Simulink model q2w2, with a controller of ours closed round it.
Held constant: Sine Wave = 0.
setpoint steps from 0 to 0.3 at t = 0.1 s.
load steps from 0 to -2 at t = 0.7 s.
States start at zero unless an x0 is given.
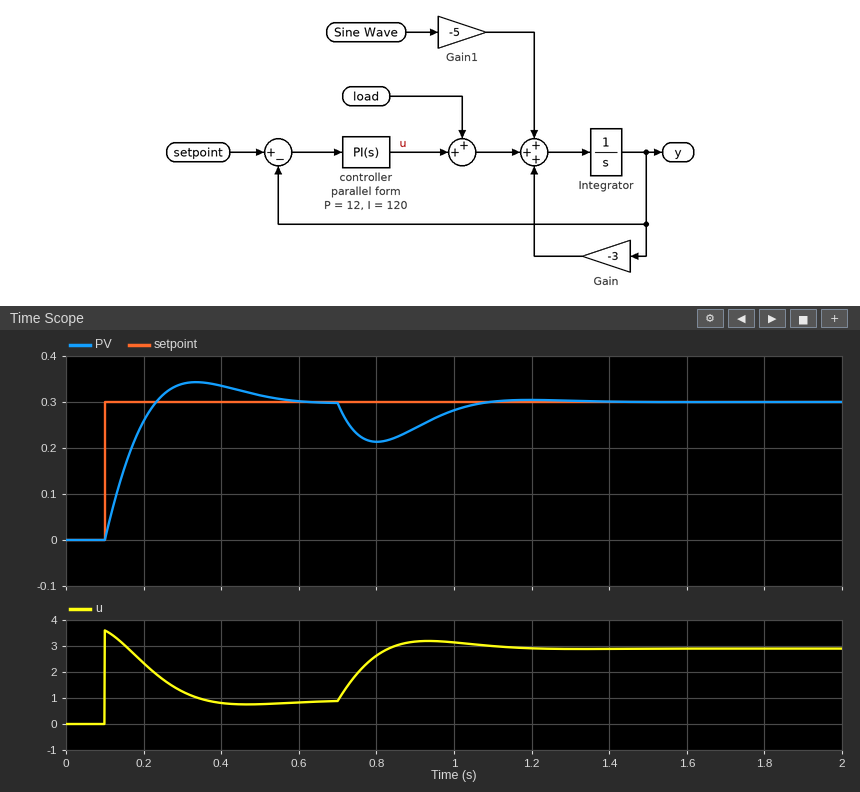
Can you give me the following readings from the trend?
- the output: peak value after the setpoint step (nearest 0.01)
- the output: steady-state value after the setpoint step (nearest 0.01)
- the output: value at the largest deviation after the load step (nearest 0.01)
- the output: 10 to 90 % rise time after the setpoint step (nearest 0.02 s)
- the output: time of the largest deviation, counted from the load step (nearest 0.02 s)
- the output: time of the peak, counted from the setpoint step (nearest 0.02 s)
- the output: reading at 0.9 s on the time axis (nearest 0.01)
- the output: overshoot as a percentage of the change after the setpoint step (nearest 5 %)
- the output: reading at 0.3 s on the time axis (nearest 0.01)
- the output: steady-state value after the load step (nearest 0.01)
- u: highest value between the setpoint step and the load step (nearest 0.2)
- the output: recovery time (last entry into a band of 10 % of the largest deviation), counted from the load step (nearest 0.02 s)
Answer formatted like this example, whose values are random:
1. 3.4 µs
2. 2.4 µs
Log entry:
1. 0.34
2. 0.30
3. 0.21
4. 0.10 s
5. 0.10 s
6. 0.24 s
7. 0.24
8. 15 %
9. 0.34
10. 0.30
11. 3.6
12. 0.34 s
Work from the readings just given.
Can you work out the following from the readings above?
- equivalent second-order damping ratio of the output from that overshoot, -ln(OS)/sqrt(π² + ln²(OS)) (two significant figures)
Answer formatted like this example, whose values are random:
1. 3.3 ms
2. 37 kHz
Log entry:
1. 0.52
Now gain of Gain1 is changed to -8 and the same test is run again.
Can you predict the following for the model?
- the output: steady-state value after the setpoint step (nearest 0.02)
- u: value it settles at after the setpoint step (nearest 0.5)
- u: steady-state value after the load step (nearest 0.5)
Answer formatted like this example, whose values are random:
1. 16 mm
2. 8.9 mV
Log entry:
1. 0.30
2. 1.0
3. 3.0
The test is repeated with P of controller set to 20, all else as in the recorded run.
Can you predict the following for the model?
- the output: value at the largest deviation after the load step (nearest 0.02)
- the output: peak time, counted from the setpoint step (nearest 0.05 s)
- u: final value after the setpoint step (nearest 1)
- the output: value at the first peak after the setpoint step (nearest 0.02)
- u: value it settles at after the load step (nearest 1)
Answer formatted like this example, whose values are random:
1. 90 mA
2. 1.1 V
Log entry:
1. 0.24
2. 0.20 s
3. 1
4. 0.32
5. 3
